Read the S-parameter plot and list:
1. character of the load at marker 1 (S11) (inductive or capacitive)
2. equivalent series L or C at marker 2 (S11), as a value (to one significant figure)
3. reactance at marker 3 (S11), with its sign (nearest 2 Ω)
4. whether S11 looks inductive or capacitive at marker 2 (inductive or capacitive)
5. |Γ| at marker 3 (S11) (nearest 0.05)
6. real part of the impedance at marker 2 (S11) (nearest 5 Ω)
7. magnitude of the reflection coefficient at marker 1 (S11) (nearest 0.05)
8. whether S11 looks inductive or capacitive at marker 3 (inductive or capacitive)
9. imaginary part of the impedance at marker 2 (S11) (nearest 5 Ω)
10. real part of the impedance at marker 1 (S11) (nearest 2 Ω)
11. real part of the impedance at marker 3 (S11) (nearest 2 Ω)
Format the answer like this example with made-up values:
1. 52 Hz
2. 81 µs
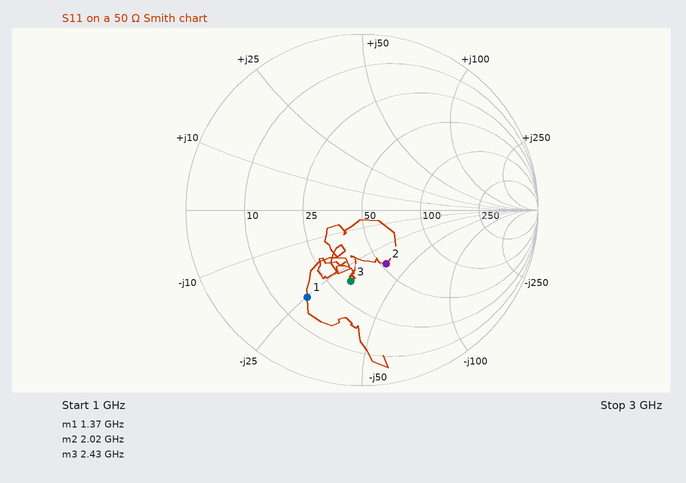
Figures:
1. capacitive
2. 2 pF
3. -32 Ω
4. capacitive
5. 0.40
6. 55 Ω
7. 0.60
8. capacitive
9. -35 Ω
10. 16 Ω
11. 32 Ω
